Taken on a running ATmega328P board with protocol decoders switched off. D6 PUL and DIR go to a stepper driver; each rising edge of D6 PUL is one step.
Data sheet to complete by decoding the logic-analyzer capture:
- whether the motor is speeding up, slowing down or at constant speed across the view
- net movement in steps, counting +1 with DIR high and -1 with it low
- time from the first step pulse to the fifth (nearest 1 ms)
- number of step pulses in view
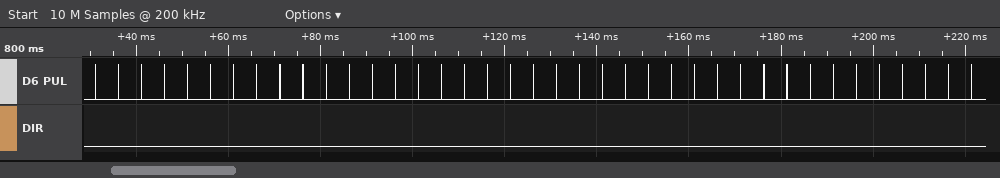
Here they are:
constant speed
-39
20 ms
39
